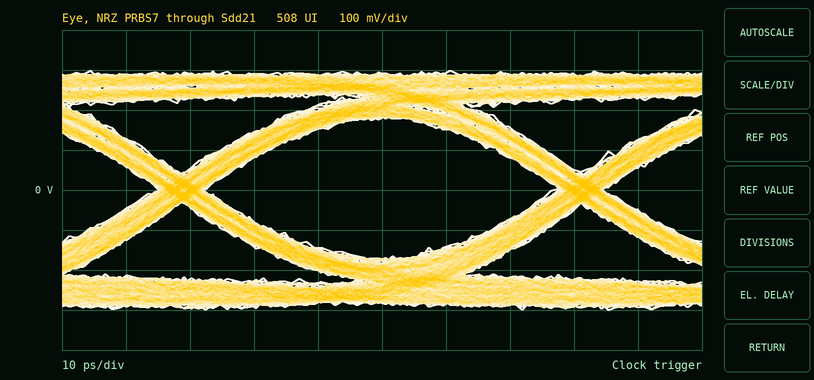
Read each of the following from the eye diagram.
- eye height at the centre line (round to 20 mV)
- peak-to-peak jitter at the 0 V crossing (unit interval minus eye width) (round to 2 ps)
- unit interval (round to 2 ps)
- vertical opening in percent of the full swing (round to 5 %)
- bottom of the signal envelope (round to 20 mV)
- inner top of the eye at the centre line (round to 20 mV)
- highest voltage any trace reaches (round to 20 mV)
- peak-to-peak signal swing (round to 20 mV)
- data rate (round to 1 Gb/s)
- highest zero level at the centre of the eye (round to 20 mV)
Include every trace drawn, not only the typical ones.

360 mV
8 ps
62 ps
60 %
-300 mV
180 mV
300 mV
600 mV
16 Gb/s
-180 mV
